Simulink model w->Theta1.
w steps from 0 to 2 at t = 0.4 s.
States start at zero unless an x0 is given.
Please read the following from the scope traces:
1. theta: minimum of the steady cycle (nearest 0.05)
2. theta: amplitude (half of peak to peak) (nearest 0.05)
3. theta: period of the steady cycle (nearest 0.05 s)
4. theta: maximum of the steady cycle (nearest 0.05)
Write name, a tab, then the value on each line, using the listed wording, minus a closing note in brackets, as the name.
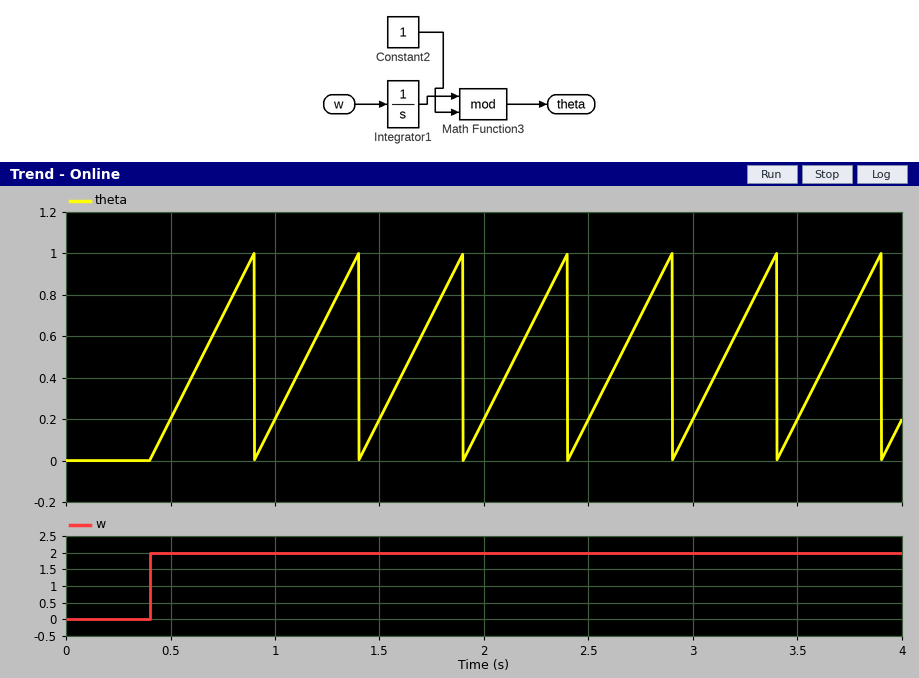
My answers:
theta: minimum of the steady cycle	0.00
theta: amplitude (half of peak to peak)	0.50
theta: period of the steady cycle	0.50 s
theta: maximum of the steady cycle	1.00
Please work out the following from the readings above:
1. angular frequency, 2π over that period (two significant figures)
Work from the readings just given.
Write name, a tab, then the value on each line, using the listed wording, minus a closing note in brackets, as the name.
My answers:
angular frequency, 2π over that period	13 rad/s
